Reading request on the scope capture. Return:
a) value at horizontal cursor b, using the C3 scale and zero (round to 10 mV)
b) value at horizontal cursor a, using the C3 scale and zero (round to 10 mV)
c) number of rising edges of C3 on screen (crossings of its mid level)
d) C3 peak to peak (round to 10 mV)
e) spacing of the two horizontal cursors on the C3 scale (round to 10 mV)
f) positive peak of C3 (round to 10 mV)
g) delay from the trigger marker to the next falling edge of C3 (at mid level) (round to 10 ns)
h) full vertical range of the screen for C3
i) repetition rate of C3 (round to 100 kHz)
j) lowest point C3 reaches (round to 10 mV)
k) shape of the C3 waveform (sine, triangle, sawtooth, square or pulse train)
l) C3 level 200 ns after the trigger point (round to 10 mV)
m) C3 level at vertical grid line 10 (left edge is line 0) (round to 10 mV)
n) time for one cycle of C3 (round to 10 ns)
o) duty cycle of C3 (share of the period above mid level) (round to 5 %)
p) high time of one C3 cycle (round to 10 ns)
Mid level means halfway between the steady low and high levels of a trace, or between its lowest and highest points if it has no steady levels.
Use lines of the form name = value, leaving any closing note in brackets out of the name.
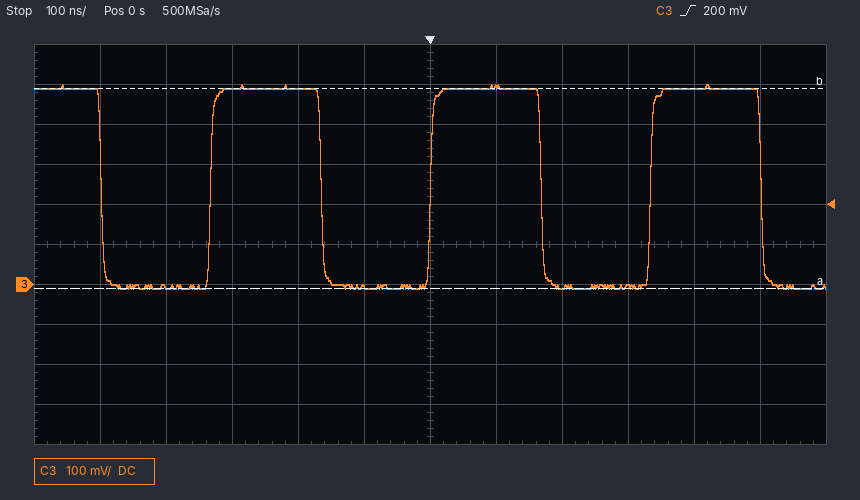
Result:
value at horizontal cursor b, using the C3 scale and zero = 490 mV
value at horizontal cursor a, using the C3 scale and zero = -10 mV
number of rising edges of C3 on screen = 3
C3 peak to peak = 510 mV
spacing of the two horizontal cursors on the C3 scale = 500 mV
positive peak of C3 = 500 mV
delay from the trigger marker to the next falling edge of C3 (at mid level) = 170 ns
full vertical range of the screen for C3 = 1 V
repetition rate of C3 = 3.0 MHz
lowest point C3 reaches = -10 mV
shape of the C3 waveform = square
C3 level 200 ns after the trigger point = -10 mV
C3 level at vertical grid line 10 (left edge is line 0) = 490 mV
time for one cycle of C3 = 330 ns
duty cycle of C3 (share of the period above mid level) = 50 %
high time of one C3 cycle = 170 ns
